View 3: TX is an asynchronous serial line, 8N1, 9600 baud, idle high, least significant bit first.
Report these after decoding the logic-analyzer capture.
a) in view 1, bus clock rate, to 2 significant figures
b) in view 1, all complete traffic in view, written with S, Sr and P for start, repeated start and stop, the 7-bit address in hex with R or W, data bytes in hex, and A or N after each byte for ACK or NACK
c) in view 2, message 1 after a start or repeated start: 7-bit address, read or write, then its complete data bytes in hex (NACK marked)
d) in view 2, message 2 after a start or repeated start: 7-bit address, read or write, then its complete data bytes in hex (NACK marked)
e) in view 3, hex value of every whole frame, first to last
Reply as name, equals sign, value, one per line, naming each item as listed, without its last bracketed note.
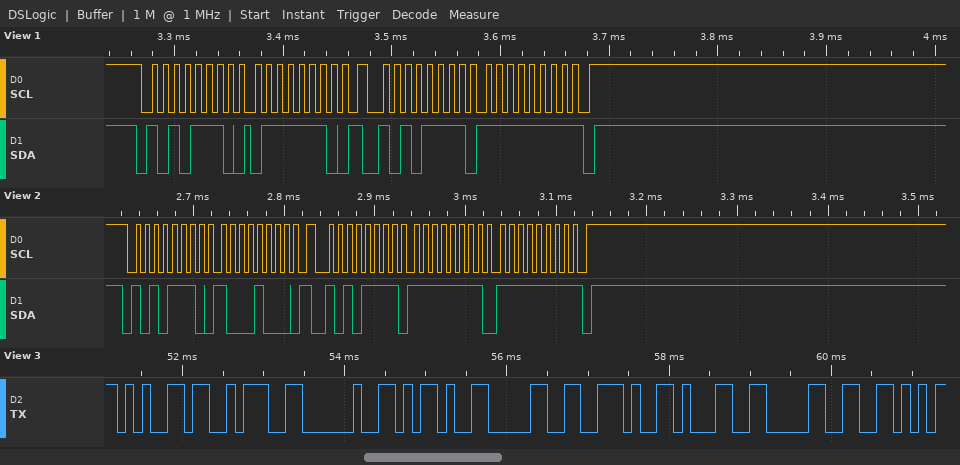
in view 1, bus clock rate, to 2 significant figures = 100 kHz
in view 1, all complete traffic in view, written with S, Sr and P for start, repeated start and stop, the 7-bit address in hex with R or W, data bytes in hex, and A or N after each byte for ACK or NACK = S 57W A 7E A Sr 57R A FF N P
in view 2, message 1 after a start or repeated start: 7-bit address, read or write, then its complete data bytes in hex = 0x57 write: 88
in view 2, message 2 after a start or repeated start: 7-bit address, read or write, then its complete data bytes in hex = 0x57 read: FF FF NACK
in view 3, hex value of every whole frame, first to last = 65 3A 20 2D 30 2E 31 30 56
